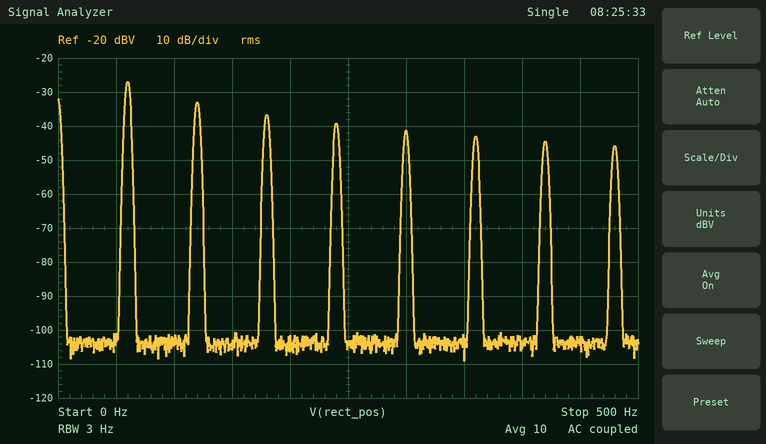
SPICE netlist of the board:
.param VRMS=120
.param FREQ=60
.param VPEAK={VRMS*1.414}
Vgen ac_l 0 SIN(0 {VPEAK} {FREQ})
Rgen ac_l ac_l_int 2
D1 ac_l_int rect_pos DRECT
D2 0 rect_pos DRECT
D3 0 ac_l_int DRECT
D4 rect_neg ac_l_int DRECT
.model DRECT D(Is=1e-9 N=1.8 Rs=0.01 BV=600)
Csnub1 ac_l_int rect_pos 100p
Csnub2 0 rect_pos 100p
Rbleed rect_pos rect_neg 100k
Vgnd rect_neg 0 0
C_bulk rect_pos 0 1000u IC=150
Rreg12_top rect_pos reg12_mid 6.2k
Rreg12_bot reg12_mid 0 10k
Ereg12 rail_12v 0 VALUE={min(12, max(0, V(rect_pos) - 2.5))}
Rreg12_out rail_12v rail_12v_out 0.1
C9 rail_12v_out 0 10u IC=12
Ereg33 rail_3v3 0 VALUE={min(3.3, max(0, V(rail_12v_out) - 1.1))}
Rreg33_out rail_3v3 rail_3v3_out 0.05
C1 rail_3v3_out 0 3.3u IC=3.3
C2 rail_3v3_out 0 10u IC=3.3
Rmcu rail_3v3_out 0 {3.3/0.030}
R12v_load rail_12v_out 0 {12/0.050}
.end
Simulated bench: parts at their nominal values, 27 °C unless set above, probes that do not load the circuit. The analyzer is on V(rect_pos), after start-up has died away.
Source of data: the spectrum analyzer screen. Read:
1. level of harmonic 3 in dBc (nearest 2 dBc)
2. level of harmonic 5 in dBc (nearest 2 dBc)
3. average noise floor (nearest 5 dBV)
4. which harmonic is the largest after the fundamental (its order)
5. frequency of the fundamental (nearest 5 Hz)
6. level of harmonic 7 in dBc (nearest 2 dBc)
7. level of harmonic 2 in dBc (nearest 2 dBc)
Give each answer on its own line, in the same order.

-10 dBc
-14 dBc
-105 dBV
2
60 Hz
-18 dBc
-6 dBc
